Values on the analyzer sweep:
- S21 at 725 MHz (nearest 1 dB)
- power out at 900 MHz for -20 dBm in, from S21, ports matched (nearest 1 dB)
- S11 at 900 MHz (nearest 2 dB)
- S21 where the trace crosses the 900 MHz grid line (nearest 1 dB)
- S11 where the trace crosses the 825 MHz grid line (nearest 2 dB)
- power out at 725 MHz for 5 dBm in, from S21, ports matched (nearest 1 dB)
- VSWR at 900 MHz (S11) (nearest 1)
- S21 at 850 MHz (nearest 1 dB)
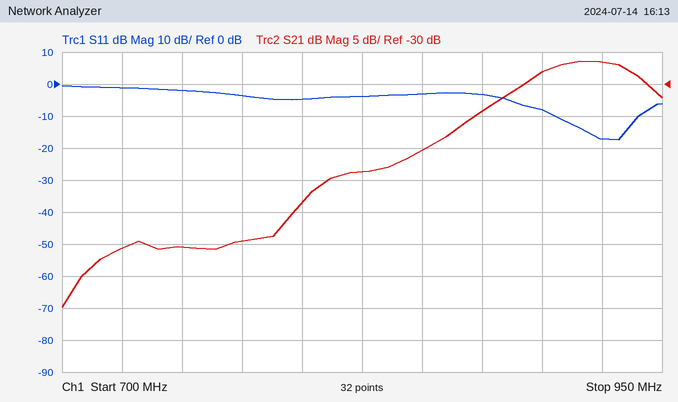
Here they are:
-56 dB
-48 dBm
-8 dB
-28 dB
-4 dB
-51 dBm
2
-40 dB
